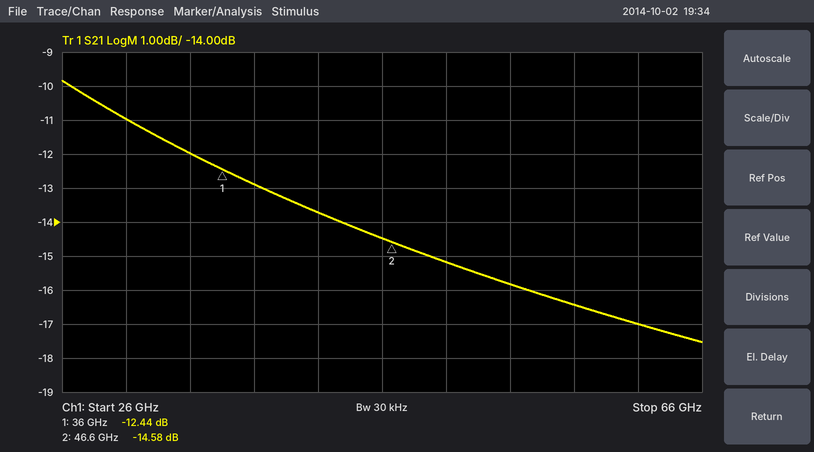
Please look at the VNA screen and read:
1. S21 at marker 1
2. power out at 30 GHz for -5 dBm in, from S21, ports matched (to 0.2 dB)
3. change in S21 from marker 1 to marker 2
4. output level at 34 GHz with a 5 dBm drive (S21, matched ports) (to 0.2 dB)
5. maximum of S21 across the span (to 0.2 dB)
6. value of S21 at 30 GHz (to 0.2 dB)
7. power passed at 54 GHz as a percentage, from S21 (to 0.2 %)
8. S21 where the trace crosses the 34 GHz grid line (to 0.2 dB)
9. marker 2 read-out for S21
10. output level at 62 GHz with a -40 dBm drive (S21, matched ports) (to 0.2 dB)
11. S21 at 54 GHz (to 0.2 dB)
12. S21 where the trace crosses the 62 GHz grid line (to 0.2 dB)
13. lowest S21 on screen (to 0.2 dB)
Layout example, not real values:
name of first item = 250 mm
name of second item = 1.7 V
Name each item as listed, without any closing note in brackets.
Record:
S21 at marker 1 = -12.44 dB
power out at 30 GHz for -5 dBm in, from S21, ports matched = -16.0 dBm
change in S21 from marker 1 to marker 2 = -2.14 dB
output level at 34 GHz with a 5 dBm drive (S21, matched ports) = -7.0 dBm
maximum of S21 across the span = -9.8 dB
value of S21 at 30 GHz = -11.0 dB
power passed at 54 GHz as a percentage, from S21 = 2.6 %
S21 where the trace crosses the 34 GHz grid line = -12.0 dB
marker 2 read-out for S21 = -14.58 dB
output level at 62 GHz with a -40 dBm drive (S21, matched ports) = -57.0 dBm
S21 at 54 GHz = -15.8 dB
S21 where the trace crosses the 62 GHz grid line = -17.0 dB
lowest S21 on screen = -17.6 dB
